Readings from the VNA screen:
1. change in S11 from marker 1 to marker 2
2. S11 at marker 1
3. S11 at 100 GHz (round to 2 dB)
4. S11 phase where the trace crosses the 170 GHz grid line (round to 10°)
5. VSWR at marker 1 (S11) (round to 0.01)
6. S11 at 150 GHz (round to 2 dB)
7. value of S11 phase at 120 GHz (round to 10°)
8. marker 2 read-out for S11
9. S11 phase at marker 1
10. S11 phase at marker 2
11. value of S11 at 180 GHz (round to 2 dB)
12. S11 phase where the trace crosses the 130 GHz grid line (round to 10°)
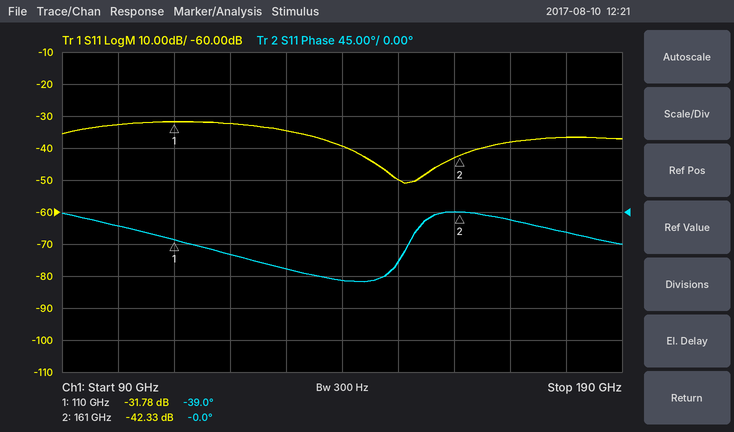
-10.55 dB
-31.78 dB
-32 dB
-10°
1.05
-50 dB
-60°
-42.33 dB
-39.0°
-0.0°
-36 dB
-80°
